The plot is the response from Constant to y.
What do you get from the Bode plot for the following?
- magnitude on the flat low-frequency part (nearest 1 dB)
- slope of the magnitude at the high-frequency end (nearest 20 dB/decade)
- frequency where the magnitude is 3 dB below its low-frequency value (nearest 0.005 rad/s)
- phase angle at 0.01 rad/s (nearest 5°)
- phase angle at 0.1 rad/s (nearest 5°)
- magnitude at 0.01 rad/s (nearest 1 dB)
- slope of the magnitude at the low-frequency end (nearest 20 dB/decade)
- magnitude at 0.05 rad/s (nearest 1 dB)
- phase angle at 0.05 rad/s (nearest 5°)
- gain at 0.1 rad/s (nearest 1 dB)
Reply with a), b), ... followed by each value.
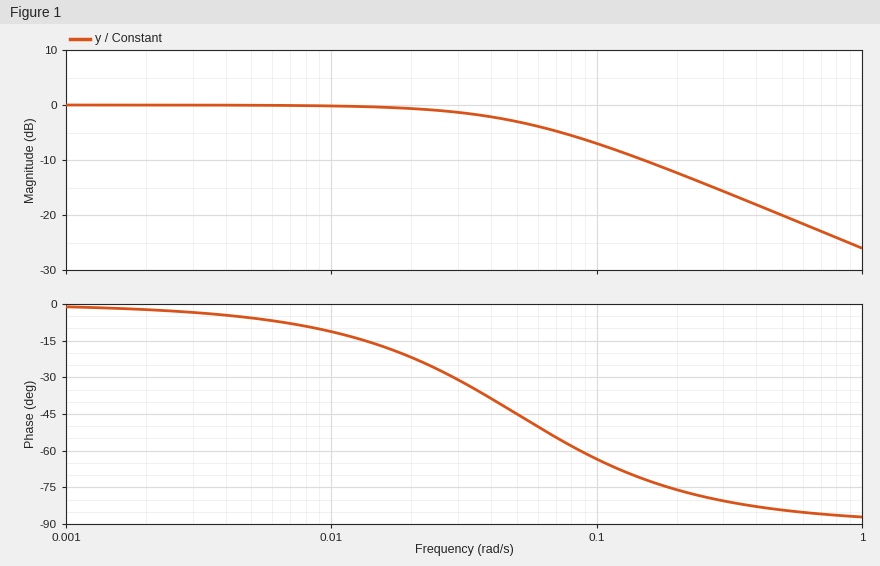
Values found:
a) 0 dB
b) -20 dB/decade
c) 0.050 rad/s
d) -10°
e) -65°
f) 0 dB
g) 0 dB/decade
h) -3 dB
i) -45°
j) -7 dB
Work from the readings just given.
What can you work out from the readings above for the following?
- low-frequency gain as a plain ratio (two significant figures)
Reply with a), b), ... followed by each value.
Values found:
a) 1.0
